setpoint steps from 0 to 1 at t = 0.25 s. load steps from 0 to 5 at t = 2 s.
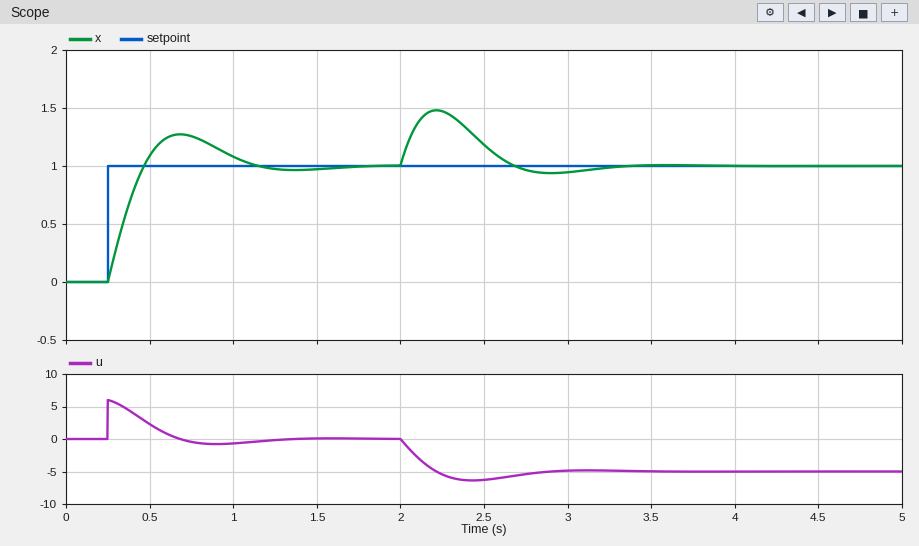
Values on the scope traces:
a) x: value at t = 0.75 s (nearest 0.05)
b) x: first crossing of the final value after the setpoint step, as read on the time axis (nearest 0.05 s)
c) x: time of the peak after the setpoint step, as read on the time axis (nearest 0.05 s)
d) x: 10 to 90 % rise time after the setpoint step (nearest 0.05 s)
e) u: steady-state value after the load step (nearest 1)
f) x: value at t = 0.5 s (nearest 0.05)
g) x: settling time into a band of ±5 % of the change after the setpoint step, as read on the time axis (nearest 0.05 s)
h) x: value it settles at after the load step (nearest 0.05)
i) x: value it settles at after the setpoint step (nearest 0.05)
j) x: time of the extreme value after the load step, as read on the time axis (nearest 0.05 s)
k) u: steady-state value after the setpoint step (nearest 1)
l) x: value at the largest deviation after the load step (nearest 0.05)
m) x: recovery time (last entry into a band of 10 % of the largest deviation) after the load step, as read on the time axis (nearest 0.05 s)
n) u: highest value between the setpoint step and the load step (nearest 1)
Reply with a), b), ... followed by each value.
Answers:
a) 1.25
b) 0.45 s
c) 0.70 s
d) 0.15 s
e) -5
f) 1.10
g) 1.05 s
h) 1.00
i) 1.00
j) 2.20 s
k) 0
l) 1.50
m) 3.05 s
n) 6
